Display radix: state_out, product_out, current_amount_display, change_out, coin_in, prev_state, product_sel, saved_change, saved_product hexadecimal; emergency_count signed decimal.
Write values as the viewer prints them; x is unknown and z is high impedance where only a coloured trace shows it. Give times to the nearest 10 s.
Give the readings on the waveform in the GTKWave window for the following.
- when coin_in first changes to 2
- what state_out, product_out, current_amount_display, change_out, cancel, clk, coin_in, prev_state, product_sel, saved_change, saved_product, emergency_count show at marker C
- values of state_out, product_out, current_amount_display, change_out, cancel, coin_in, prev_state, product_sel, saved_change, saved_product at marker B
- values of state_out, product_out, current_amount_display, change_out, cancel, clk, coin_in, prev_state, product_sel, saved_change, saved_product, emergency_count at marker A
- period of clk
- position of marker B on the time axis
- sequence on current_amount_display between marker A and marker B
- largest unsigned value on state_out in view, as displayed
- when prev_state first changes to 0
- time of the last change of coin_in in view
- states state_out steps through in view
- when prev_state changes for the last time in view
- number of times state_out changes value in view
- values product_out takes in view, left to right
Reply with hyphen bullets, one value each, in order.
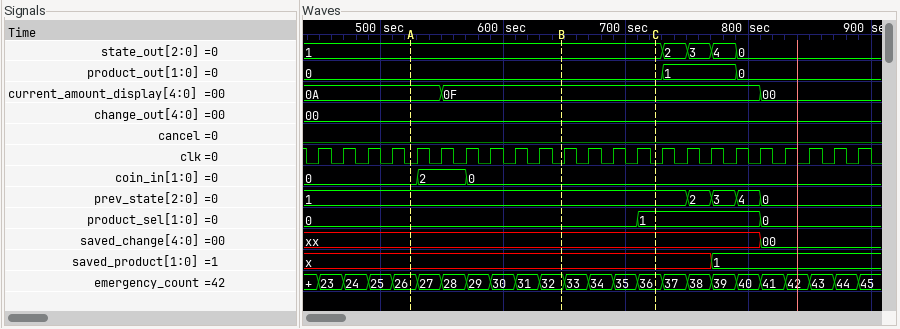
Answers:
- 530 s
- state_out=1, product_out=0, current_amount_display=0F, change_out=00, cancel=0, clk=0, coin_in=0, prev_state=1, product_sel=1, saved_change=xx, saved_product=x, emergency_count=36
- state_out=1, product_out=0, current_amount_display=0F, change_out=00, cancel=0, coin_in=0, prev_state=1, product_sel=0, saved_change=xx, saved_product=x
- state_out=1, product_out=0, current_amount_display=0A, change_out=00, cancel=0, clk=0, coin_in=0, prev_state=1, product_sel=0, saved_change=xx, saved_product=x, emergency_count=26
- 20 s
- 650 s
- 0A, 0F
- 4
- 810 s
- 570 s
- 1, 2, 3, 4, 0
- 810 s
- 4
- 0, 1, 0
